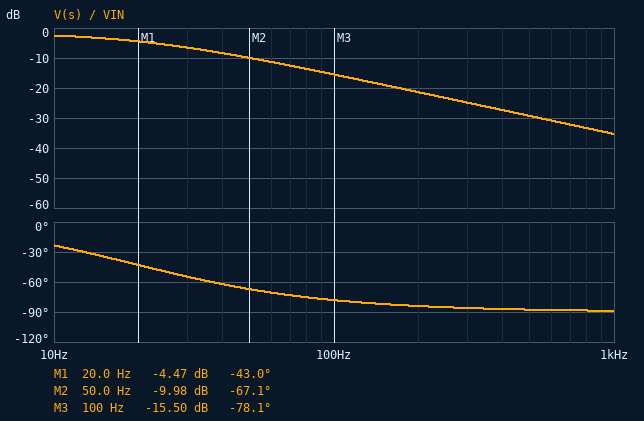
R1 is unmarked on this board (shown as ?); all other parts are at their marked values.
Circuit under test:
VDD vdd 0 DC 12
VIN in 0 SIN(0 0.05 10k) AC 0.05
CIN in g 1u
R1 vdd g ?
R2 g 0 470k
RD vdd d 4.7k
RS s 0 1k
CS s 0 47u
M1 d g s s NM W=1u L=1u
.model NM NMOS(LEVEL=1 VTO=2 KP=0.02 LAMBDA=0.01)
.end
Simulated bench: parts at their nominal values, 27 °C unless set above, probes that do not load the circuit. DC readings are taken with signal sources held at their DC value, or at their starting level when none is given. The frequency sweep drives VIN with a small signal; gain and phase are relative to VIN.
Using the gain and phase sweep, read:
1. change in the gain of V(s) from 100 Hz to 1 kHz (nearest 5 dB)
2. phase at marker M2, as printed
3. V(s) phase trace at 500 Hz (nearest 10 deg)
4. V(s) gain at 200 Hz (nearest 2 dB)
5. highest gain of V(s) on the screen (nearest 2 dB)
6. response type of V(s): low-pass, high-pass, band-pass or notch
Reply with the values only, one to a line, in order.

-20 dB
-67.1 deg
-90 deg
-22 dB
-2 dB
low-pass
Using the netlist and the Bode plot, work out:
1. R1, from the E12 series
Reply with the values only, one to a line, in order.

1.5 MΩ
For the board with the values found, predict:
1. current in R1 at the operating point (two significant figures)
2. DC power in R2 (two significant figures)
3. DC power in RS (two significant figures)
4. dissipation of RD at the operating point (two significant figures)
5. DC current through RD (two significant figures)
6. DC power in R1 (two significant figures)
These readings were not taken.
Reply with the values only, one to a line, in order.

6.1 µA
17 µW
390 µW
1.8 mW
620 µA
56 µW
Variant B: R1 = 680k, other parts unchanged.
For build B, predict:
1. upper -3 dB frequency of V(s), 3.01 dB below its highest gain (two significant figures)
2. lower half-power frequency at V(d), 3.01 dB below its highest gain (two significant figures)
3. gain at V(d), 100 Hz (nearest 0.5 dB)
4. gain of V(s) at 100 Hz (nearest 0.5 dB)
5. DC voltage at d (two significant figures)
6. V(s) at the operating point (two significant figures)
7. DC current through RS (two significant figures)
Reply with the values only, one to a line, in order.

5.3 Hz
1.0 Hz
-14.0 dB
-57.0 dB
2.2 V
2.1 V
2.1 mA
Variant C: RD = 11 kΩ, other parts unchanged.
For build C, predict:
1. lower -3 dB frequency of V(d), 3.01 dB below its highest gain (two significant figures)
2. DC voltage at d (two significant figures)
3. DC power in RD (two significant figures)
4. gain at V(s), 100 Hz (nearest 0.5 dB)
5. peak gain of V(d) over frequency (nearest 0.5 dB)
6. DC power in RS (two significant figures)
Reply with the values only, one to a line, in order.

19 Hz
5.2 V
4.2 mW
-16.0 dB
34.5 dB
380 µW
